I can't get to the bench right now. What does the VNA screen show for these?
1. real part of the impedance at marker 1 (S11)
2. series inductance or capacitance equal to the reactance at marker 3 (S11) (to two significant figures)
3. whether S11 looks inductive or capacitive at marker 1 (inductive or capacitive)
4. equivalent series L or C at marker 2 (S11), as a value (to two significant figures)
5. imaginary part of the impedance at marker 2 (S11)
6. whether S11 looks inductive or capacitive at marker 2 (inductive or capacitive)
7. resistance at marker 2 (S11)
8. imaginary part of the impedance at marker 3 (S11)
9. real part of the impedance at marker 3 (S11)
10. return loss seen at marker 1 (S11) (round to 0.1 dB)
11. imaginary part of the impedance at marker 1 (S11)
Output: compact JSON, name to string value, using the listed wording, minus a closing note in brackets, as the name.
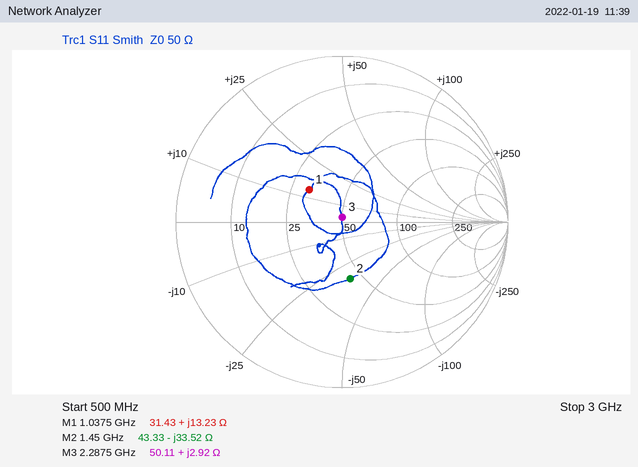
{"real part of the impedance at marker 1": "31.43 Ω", "series inductance or capacitance equal to the reactance at marker 3 (S11)": "200 pH", "whether S11 looks inductive or capacitive at marker 1": "inductive", "equivalent series L or C at marker 2 (S11), as a value": "3.3 pF", "imaginary part of the impedance at marker 2": "-33.52 Ω", "whether S11 looks inductive or capacitive at marker 2": "capacitive", "resistance at marker 2": "43.33 Ω", "imaginary part of the impedance at marker 3": "+2.92 Ω", "real part of the impedance at marker 3": "50.11 Ω", "return loss seen at marker 1 (S11)": "11.2 dB", "imaginary part of the impedance at marker 1": "+13.23 Ω"}
